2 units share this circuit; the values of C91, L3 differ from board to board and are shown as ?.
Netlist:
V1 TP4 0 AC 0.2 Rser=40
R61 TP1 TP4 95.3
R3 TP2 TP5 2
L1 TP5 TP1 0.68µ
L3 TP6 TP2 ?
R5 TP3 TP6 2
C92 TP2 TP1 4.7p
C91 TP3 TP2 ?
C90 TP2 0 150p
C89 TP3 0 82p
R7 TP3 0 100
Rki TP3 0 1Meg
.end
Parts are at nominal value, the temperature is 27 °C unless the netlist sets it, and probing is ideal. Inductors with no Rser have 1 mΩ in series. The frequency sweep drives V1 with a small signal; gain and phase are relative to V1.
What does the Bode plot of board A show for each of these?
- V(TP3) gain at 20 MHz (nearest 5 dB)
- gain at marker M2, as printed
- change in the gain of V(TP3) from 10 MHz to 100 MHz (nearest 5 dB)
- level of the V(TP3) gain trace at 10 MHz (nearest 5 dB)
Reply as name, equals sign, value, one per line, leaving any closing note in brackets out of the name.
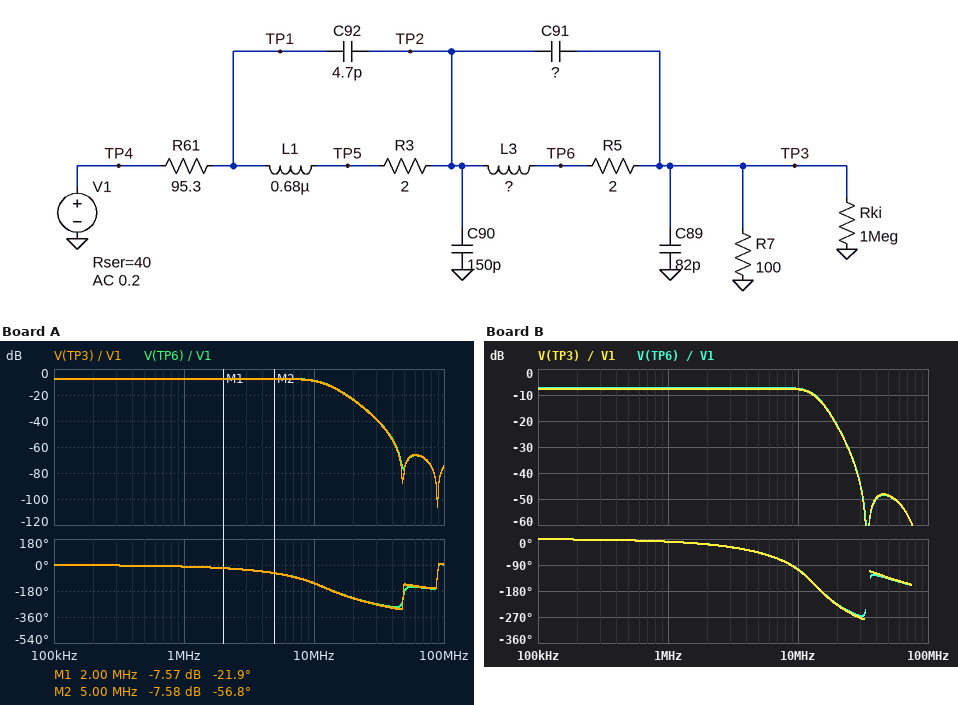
V(TP3) gain at 20 MHz = -25 dB
gain at marker M2, as printed = -7.58 dB
change in the gain of V(TP3) from 10 MHz to 100 MHz = -65 dB
level of the V(TP3) gain trace at 10 MHz = -10 dB
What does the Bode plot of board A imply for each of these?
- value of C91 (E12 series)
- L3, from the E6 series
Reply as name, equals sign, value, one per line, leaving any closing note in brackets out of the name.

value of C91 = 3.3 pF
L3, from the E6 series = 3.3 µH
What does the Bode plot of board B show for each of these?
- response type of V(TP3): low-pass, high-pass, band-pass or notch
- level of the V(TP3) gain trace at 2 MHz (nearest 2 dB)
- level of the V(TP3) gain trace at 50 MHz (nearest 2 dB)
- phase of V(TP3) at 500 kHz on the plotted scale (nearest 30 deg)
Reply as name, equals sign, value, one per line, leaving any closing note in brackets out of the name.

response type of V(TP3): low-pass, high-pass, band-pass or notch = low-pass
level of the V(TP3) gain trace at 2 MHz = -8 dB
level of the V(TP3) gain trace at 50 MHz = -48 dB
phase of V(TP3) at 500 kHz on the plotted scale = 0 deg
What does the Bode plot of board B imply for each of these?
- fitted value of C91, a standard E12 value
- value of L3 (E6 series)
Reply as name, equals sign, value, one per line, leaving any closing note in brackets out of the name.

fitted value of C91, a standard E12 value = 10 pF
value of L3 = 2.2 µH
